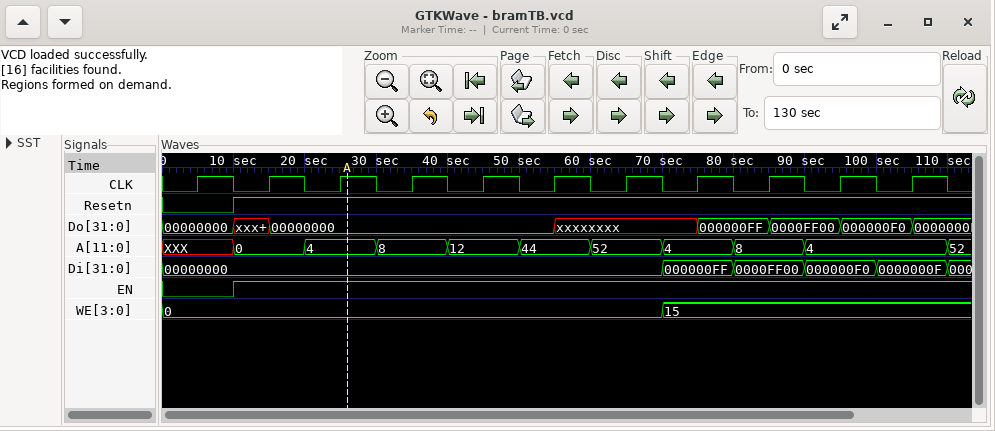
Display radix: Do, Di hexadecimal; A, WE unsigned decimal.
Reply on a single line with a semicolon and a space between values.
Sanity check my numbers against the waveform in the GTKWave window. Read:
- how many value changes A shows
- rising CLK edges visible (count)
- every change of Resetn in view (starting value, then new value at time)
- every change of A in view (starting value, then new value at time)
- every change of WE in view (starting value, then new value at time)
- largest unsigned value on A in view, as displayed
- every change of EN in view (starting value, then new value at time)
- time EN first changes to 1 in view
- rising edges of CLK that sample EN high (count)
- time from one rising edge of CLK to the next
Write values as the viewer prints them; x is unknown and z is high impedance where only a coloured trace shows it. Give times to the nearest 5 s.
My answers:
10; 11; 0, 1 at 10 s; XXX, 0 at 10 s, 4 at 20 s, 8 at 30 s, 12 at 40 s, 44 at 50 s, 52 at 60 s, 4 at 70 s, 8 at 80 s, 4 at 90 s, 52 at 110 s; 0, 15 at 70 s; 52; 0, 1 at 10 s; 10 s; 10; 10 s
